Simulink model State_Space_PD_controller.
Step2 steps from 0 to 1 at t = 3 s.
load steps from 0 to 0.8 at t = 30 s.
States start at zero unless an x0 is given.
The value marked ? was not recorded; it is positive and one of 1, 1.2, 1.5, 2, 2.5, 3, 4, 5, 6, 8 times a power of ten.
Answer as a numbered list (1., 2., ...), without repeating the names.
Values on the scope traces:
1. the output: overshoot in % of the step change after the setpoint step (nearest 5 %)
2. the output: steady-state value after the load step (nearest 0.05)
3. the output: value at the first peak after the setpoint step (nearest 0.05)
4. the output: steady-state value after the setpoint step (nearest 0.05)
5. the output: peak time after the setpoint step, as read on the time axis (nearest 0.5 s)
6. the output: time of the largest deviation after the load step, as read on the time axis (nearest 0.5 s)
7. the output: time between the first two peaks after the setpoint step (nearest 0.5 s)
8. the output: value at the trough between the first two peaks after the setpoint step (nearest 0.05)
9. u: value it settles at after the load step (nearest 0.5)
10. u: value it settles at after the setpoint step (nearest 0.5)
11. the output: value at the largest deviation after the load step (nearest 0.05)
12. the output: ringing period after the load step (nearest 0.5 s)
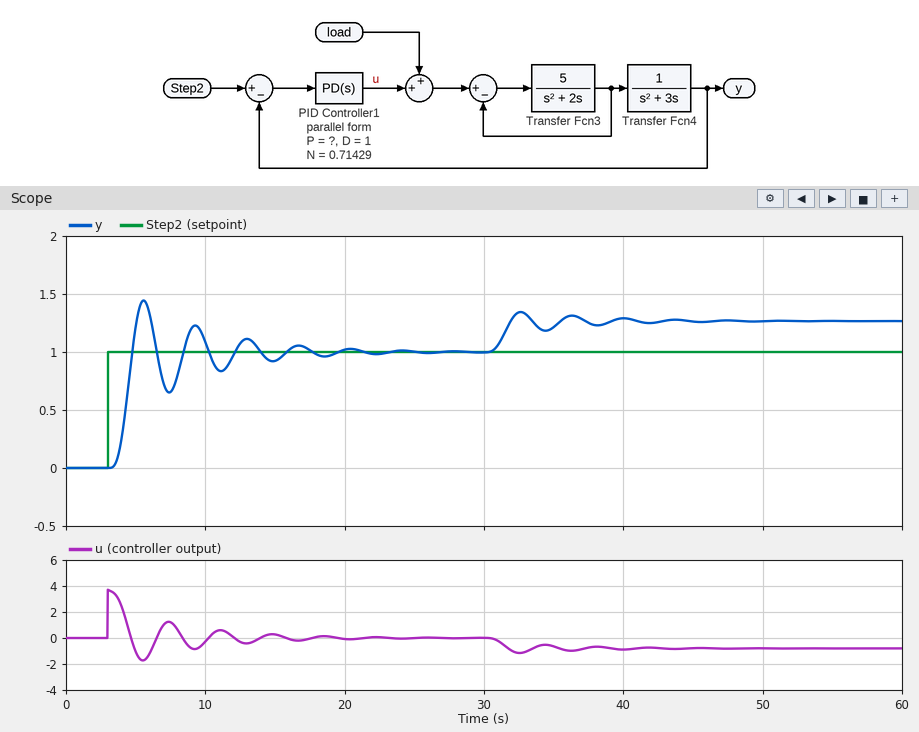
1. 45 %
2. 1.25
3. 1.45
4. 1.00
5. 5.5 s
6. 32.5 s
7. 3.5 s
8. 0.65
9. -1.0
10. 0.0
11. 1.35
12. 3.5 s
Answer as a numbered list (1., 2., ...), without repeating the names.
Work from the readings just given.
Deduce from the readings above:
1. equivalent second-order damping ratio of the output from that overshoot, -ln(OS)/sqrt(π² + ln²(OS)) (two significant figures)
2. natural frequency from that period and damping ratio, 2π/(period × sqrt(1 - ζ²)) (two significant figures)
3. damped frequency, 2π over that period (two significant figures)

1. 0.25
2. 1.9 rad/s
3. 1.8 rad/s
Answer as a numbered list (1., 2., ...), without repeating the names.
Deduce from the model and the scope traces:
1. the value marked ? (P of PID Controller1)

1. 3
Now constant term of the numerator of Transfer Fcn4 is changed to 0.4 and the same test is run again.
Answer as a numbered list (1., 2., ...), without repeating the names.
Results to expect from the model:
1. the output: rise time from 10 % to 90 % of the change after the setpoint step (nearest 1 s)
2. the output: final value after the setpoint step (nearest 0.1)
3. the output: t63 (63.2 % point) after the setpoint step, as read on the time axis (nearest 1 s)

1. 4 s
2. 1.0
3. 5 s
